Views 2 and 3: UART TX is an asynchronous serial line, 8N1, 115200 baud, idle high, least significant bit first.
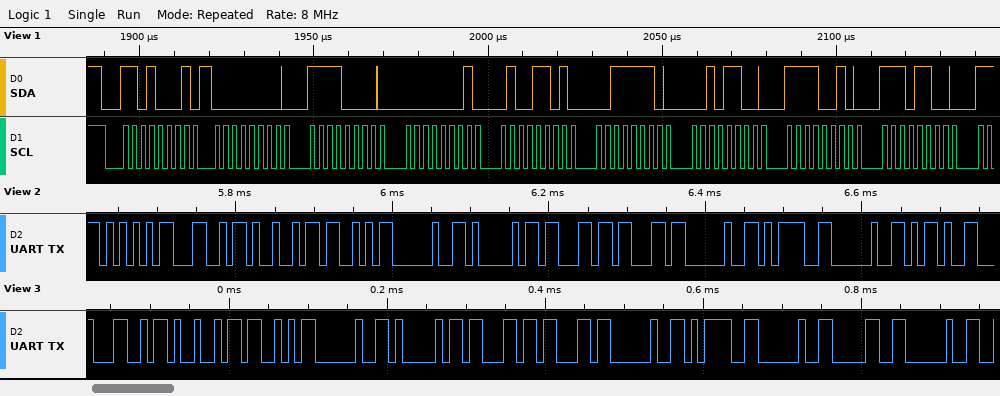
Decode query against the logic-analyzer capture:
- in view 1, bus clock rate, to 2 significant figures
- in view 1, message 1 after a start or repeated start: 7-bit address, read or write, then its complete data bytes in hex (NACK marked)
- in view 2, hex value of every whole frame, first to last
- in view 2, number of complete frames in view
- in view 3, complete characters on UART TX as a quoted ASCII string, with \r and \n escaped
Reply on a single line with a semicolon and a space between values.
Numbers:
400 kHz; 0x68 read: 00 F0 01 4D 3E 2C F2 EC; 55 4C 49 53 20 41 63 63 20 3D 20 2D; 12; "LIS Acc = 0 "
